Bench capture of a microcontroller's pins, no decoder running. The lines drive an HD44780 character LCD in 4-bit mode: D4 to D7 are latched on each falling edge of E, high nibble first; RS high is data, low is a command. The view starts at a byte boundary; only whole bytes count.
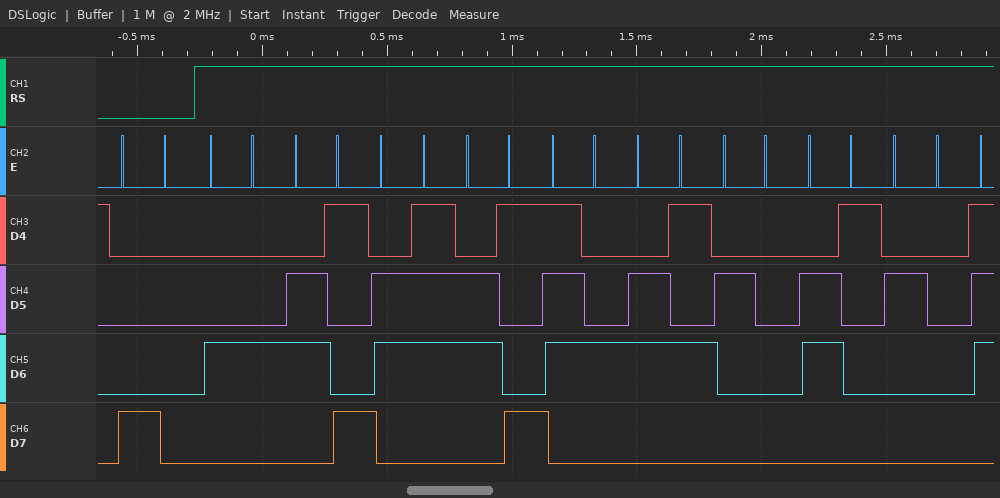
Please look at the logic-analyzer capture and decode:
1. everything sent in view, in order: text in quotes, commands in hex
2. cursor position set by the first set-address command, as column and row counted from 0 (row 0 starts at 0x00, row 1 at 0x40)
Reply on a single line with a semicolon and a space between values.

0x80 "Digite a "; column 0, row 0
